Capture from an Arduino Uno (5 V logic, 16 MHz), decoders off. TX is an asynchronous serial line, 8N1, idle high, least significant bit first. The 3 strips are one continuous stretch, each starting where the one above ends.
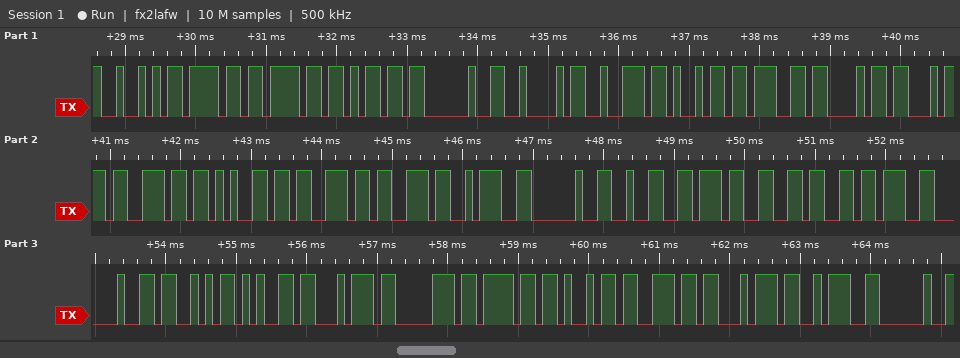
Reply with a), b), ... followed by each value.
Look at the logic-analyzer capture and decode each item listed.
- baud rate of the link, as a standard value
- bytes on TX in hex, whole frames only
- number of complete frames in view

a) 9600 baud
b) 52 6F 6F 6D 20 42 72 69 67 68 74 6E 65 73 73 3A 20 32 37 36 3B 20 53 65 74 70 6F 69 6E 74 3A 20
c) 32
